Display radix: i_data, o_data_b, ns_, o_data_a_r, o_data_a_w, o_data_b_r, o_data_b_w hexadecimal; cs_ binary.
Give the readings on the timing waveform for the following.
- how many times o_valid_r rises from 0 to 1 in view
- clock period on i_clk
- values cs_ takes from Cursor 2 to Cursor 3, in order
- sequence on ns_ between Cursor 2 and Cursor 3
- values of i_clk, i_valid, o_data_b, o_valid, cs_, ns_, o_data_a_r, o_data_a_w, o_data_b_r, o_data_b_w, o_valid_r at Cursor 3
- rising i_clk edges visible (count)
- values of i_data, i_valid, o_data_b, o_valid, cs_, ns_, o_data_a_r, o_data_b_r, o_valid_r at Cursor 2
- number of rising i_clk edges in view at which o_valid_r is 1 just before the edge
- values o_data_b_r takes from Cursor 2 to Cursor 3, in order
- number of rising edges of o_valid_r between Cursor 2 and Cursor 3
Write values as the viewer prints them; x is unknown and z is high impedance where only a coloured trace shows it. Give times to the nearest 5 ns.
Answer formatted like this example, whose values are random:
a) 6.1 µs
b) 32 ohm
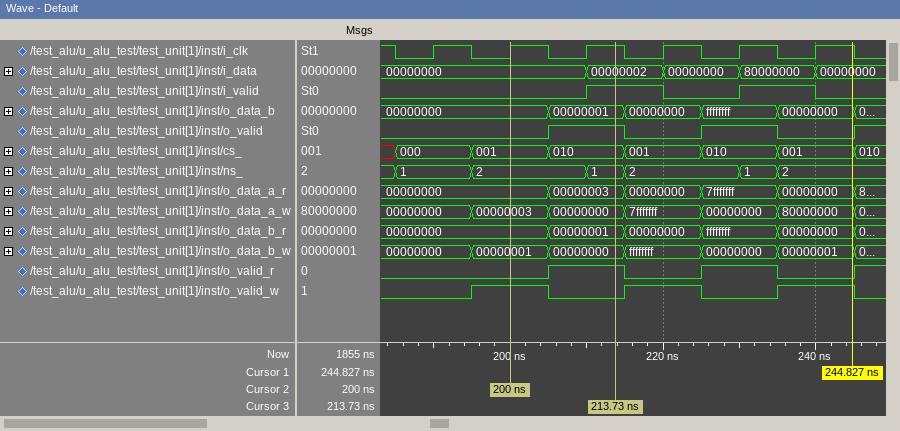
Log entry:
a) 3
b) 10 ns
c) 001, 010
d) 2, 1
e) i_clk=1, i_valid=1, o_data_b=00000001, o_valid=1, cs_=010, ns_=1, o_data_a_r=00000003, o_data_a_w=00000000, o_data_b_r=00000001, o_data_b_w=00000000, o_valid_r=1
f) 6
g) i_data=00000000, i_valid=0, o_data_b=00000000, o_valid=0, cs_=001, ns_=2, o_data_a_r=00000000, o_data_b_r=00000000, o_valid_r=0
h) 2
i) 00000000, 00000001
j) 1
